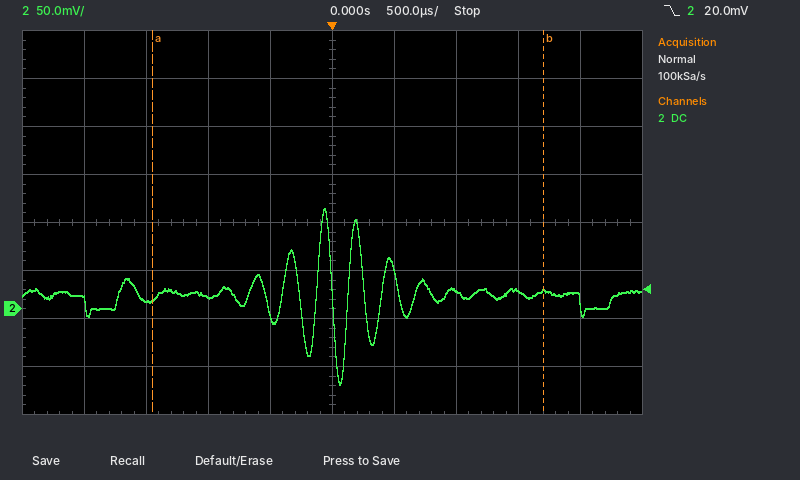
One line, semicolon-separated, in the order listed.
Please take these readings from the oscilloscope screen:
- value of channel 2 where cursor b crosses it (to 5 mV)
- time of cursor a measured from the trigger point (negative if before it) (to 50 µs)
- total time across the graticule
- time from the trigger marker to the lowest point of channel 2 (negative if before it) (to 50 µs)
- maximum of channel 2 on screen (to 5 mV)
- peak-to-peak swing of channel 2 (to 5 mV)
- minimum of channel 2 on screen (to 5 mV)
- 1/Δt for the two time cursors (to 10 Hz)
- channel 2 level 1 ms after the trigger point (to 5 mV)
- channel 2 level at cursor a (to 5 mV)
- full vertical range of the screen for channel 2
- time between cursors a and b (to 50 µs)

20 mV; -1.45 ms; 5 ms; +50 µs; 105 mV; 185 mV; -80 mV; 320 Hz; 20 mV; 10 mV; 400 mV; 3.15 ms
